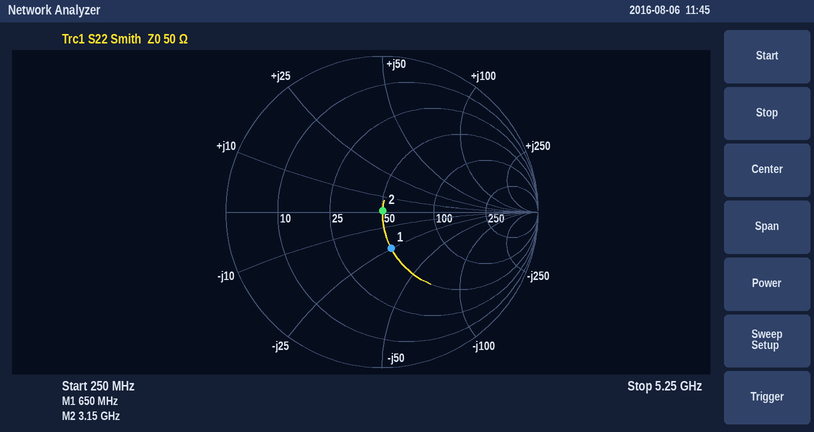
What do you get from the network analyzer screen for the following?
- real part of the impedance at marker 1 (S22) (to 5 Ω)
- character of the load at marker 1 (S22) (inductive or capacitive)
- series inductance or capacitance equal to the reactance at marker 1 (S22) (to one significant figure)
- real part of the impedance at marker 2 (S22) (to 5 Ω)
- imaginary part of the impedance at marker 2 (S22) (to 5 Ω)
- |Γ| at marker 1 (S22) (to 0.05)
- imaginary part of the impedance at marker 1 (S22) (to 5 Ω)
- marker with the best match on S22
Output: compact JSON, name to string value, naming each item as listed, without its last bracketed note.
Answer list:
{"real part of the impedance at marker 1 (S22)": "50 Ω", "character of the load at marker 1 (S22)": "capacitive", "series inductance or capacitance equal to the reactance at marker 1 (S22)": "10 pF", "real part of the impedance at marker 2 (S22)": "50 Ω", "imaginary part of the impedance at marker 2 (S22)": "0 Ω", "|Γ| at marker 1 (S22)": "0.25", "imaginary part of the impedance at marker 1 (S22)": "-25 Ω", "marker with the best match on S22": "marker 2"}
